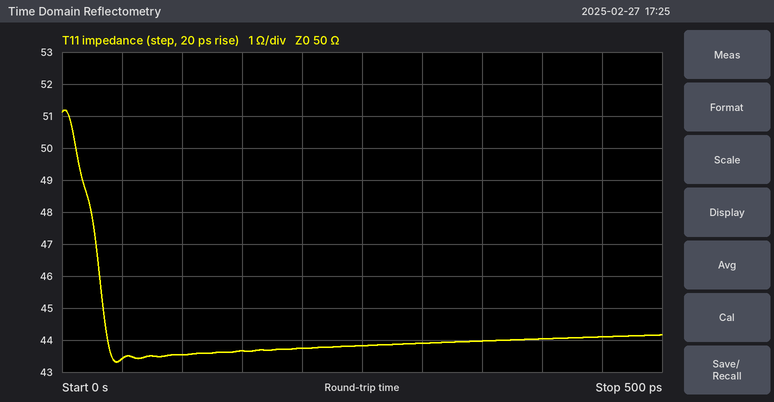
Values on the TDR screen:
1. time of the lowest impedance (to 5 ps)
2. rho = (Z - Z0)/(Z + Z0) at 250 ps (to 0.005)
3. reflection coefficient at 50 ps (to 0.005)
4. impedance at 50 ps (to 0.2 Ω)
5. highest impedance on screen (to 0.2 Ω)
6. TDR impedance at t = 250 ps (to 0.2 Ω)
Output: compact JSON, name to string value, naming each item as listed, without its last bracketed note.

{"time of the lowest impedance": "45 ps", "rho = (Z - Z0)/(Z + Z0) at 250 ps": "-0.065", "reflection coefficient at 50 ps": "-0.070", "impedance at 50 ps": "43.4 Ω", "highest impedance on screen": "51.2 Ω", "TDR impedance at t = 250 ps": "43.8 Ω"}
